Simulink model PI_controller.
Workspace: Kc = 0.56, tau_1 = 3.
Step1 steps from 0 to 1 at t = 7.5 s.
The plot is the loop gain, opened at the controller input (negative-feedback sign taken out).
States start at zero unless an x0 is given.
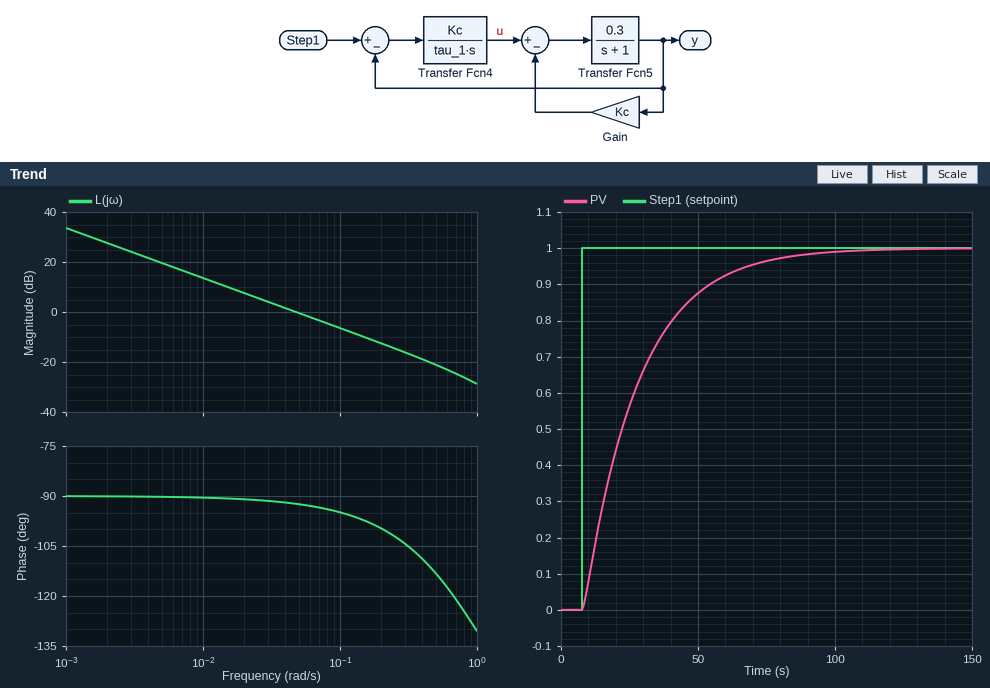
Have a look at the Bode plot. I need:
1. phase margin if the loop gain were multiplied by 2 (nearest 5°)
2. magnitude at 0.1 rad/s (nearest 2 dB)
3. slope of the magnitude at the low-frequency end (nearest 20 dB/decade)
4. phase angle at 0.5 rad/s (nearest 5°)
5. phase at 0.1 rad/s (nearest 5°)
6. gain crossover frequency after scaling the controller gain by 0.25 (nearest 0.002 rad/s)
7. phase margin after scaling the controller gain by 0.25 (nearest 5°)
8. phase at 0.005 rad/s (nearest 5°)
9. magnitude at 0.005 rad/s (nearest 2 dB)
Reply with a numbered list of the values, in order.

1. 85°
2. -6 dB
3. -20 dB/decade
4. -115°
5. -95°
6. 0.012 rad/s
7. 90°
8. -90°
9. 20 dB
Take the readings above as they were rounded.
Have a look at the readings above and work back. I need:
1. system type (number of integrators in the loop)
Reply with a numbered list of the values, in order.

1. 1
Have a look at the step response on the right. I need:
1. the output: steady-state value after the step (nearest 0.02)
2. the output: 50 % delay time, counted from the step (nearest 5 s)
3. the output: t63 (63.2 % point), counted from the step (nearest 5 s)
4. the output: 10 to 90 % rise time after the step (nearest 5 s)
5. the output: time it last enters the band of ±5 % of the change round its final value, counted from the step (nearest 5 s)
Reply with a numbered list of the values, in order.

1. 1.00
2. 15 s
3. 20 s
4. 45 s
5. 60 s
